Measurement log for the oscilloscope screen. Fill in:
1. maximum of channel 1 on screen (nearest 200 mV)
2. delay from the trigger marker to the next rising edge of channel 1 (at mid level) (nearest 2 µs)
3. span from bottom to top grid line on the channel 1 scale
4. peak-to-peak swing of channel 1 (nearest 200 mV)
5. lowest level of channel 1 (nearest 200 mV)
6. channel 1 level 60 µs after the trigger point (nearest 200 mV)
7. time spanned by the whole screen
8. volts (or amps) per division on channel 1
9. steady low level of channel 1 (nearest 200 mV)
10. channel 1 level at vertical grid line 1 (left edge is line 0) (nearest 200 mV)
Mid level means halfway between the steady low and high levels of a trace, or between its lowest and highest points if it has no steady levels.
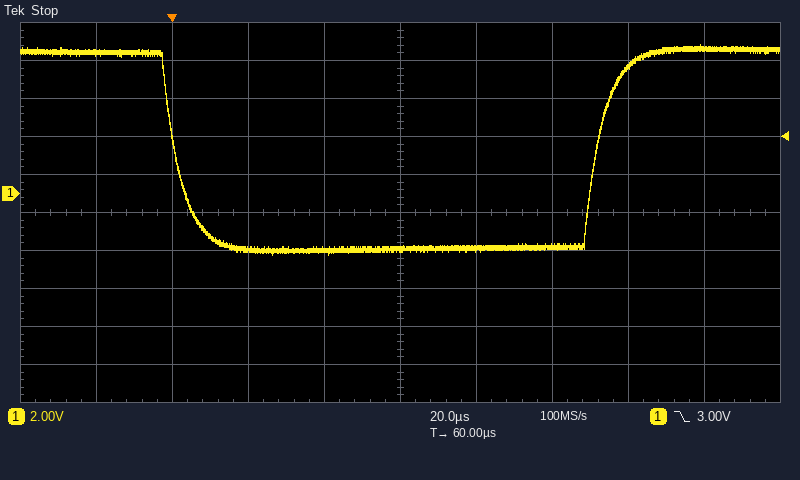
7.8 V
112 µs
20 V
11.0 V
-3.2 V
-2.8 V
200 µs
2 V
-2.8 V
7.4 V
